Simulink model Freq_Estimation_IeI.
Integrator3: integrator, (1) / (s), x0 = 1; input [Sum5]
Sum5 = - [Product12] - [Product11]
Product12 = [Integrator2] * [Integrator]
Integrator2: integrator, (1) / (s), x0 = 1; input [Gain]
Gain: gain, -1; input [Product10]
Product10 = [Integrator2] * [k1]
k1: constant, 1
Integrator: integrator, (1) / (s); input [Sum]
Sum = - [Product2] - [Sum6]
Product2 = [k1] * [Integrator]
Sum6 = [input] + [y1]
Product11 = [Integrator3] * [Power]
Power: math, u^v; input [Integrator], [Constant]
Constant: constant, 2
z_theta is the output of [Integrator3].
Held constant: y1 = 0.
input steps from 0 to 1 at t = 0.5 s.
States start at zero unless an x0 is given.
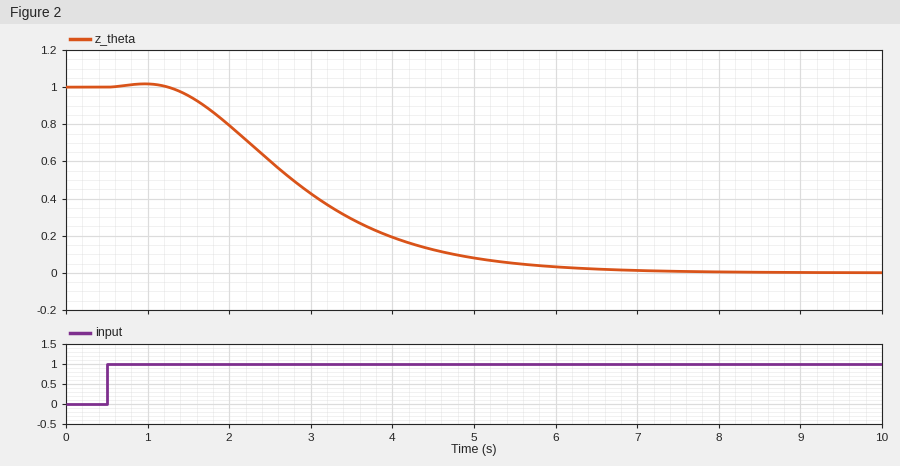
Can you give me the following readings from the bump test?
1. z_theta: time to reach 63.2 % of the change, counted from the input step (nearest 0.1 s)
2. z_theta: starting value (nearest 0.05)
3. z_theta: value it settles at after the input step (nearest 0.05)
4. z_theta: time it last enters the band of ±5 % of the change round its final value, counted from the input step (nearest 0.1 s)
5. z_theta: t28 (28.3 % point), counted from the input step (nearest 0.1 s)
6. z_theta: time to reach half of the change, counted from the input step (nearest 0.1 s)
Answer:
2.7 s
1.00
0.00
5.0 s
1.7 s
2.3 s
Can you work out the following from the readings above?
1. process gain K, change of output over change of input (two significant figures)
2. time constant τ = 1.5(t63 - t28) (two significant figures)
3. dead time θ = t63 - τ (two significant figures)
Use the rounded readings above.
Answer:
-1.0
1.5 s
1.2 s
